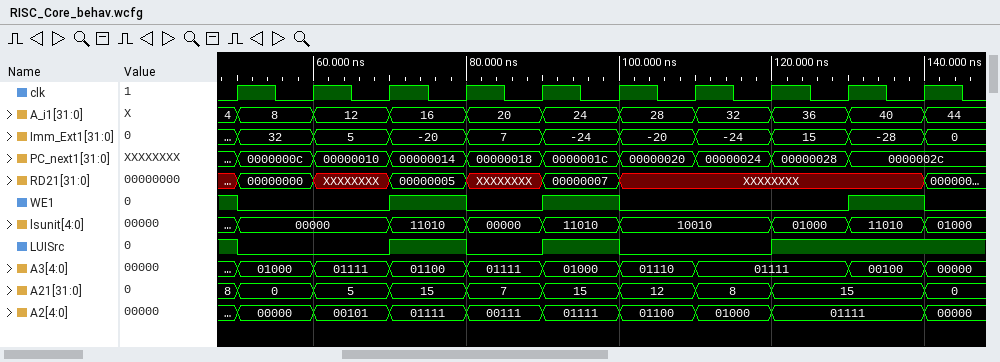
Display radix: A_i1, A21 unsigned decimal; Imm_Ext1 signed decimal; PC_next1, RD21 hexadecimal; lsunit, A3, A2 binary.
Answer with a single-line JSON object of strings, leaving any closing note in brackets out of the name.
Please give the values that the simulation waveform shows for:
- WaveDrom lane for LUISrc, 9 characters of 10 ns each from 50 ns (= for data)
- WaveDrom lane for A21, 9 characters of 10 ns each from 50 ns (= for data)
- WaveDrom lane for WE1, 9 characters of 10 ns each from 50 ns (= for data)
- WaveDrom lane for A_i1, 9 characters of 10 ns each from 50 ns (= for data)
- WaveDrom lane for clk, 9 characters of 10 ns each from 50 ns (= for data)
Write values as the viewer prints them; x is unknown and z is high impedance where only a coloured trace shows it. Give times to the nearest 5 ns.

{"WaveDrom lane for LUISrc, 9 characters of 10 ns each from 50 ns": "{name: 'LUISrc', wave: '0.1010.1.'}", "WaveDrom lane for A21, 9 characters of 10 ns each from 50 ns": "{name: 'A21', wave: '========.', data: '0 5 15 7 15 12 8 15'}", "WaveDrom lane for WE1, 9 characters of 10 ns each from 50 ns": "{name: 'WE1', wave: '0.1010..1'}", "WaveDrom lane for A_i1, 9 characters of 10 ns each from 50 ns": "{name: 'A_i1', wave: '=========', data: '8 12 16 20 24 28 32 36 40'}", "WaveDrom lane for clk, 9 characters of 10 ns each from 50 ns": "{name: 'clk', wave: 'p........'}"}
